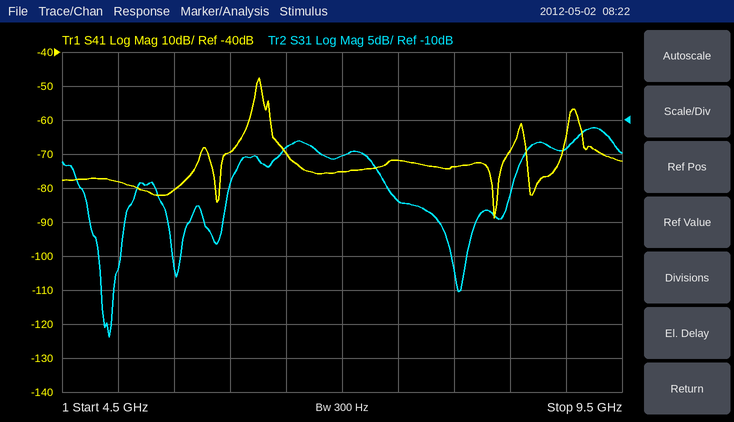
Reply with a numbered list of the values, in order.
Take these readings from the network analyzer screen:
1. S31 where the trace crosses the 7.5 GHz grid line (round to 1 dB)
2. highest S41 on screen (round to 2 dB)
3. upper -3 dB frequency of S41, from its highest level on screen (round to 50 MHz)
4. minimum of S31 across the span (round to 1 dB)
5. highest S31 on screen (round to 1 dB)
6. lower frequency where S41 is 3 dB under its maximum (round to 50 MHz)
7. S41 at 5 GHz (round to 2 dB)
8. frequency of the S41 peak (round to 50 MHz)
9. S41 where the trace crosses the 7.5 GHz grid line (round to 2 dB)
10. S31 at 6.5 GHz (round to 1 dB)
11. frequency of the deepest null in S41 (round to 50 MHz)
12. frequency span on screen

1. -22 dB
2. -48 dB
3. 6.30 GHz
4. -42 dB
5. -11 dB
6. 6.25 GHz
7. -78 dB
8. 6.25 GHz
9. -72 dB
10. -14 dB
11. 8.35 GHz
12. 5 GHz
